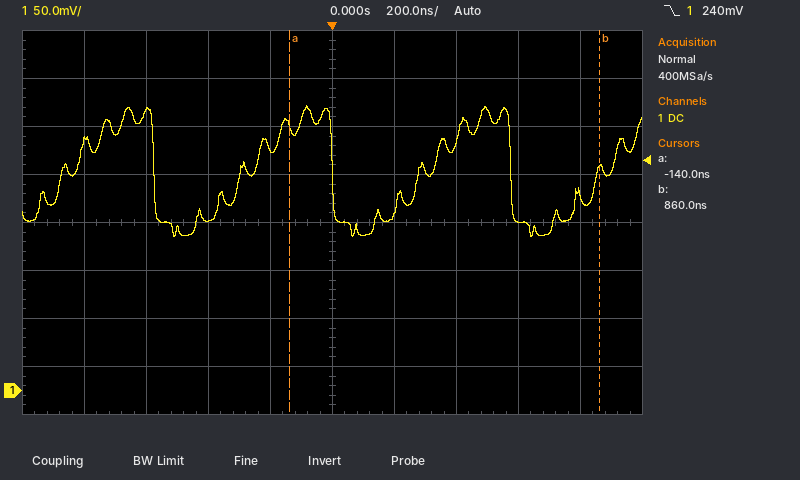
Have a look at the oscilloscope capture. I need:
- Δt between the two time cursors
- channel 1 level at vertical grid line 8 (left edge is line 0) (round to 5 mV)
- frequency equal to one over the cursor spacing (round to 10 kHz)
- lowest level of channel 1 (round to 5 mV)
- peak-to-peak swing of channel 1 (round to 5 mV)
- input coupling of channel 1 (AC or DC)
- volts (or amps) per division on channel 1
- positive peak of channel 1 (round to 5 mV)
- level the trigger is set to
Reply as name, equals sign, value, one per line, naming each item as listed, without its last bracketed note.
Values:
Δt between the two time cursors = 1.00 µs
channel 1 level at vertical grid line 8 (left edge is line 0) = 175 mV
frequency equal to one over the cursor spacing = 1.00 MHz
lowest level of channel 1 = 160 mV
peak-to-peak swing of channel 1 = 135 mV
input coupling of channel 1 = DC
volts (or amps) per division on channel 1 = 50 mV
positive peak of channel 1 = 295 mV
level the trigger is set to = 240 mV
